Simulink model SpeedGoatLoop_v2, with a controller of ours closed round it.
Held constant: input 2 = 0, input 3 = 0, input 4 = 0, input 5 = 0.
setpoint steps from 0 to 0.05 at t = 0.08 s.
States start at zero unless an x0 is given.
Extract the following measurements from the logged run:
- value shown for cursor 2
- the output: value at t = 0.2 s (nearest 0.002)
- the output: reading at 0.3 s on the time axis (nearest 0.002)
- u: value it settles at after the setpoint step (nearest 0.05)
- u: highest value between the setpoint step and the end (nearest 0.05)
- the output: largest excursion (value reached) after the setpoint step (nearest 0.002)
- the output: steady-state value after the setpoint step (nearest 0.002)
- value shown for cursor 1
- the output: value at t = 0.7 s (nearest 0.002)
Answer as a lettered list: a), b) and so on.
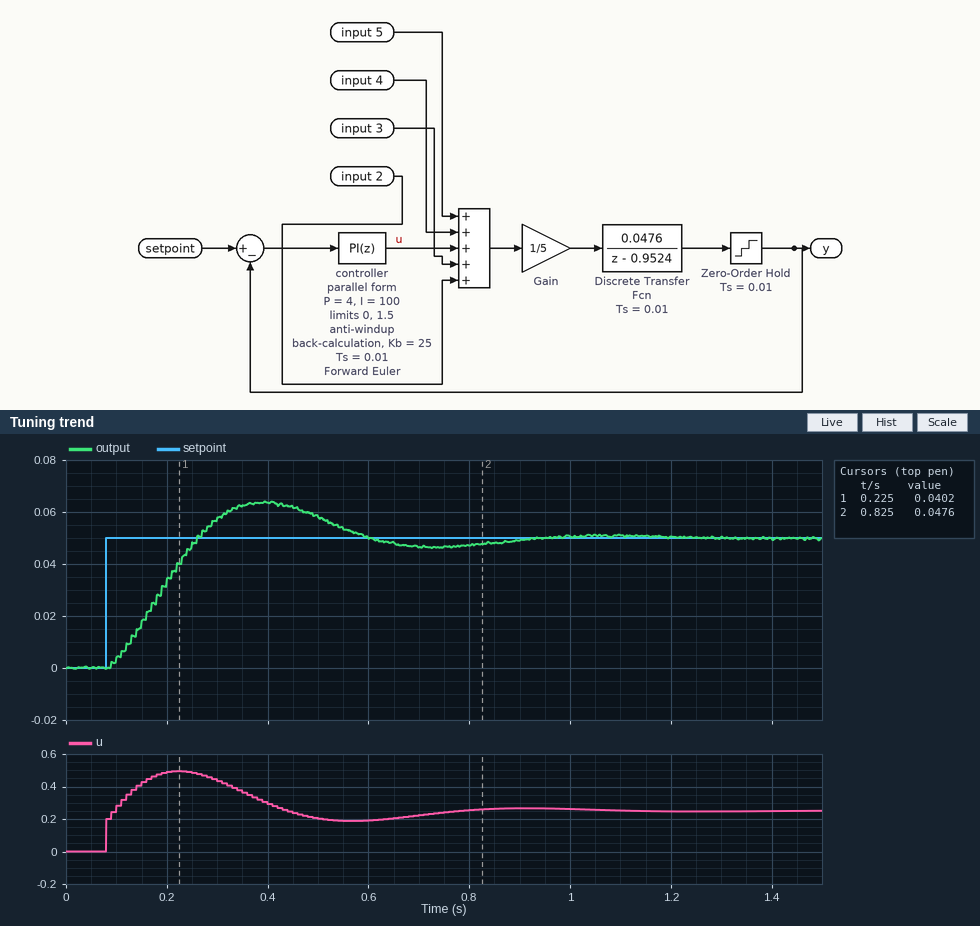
a) 0.0476
b) 0.034
c) 0.058
d) 0.25
e) 0.50
f) 0.064
g) 0.050
h) 0.0402
i) 0.046
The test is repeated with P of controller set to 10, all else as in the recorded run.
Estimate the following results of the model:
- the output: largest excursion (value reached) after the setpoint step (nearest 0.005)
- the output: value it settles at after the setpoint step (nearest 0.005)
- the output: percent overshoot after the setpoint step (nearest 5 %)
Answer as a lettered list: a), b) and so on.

a) 0.055
b) 0.050
c) 10 %
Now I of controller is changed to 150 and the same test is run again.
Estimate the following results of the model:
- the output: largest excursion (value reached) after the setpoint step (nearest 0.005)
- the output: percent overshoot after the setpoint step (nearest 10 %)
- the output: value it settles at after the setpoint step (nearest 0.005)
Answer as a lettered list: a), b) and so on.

a) 0.070
b) 40 %
c) 0.050
